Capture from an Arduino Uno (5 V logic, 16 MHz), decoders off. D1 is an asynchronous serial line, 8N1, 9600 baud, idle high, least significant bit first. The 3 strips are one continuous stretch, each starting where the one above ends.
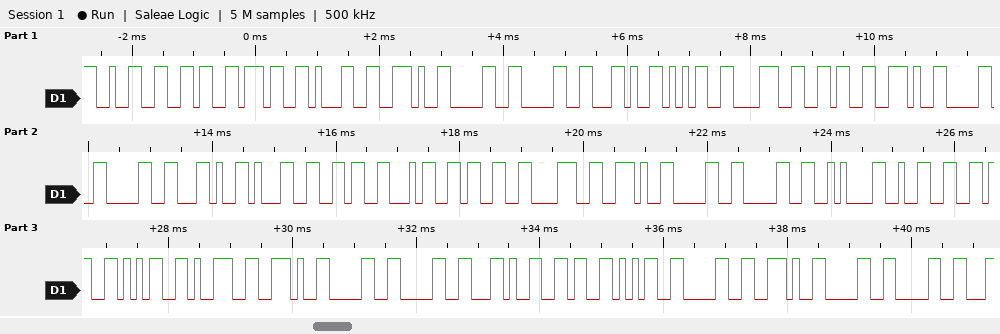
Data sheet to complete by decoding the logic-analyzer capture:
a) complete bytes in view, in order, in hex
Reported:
0x32 0x36 0x37 0x31 0x2E 0x30 0x30 0x2C 0x35 0x38 0x36 0x2E 0x30 0x30 0x2C 0x31 0x36 0x34 0x33 0x38 0x2E 0x30 0x30 0x0A 0x32 0x36 0x35 0x39 0x2E 0x30 0x30 0x2C 0x36 0x35 0x30 0x2E 0x30 0x30
